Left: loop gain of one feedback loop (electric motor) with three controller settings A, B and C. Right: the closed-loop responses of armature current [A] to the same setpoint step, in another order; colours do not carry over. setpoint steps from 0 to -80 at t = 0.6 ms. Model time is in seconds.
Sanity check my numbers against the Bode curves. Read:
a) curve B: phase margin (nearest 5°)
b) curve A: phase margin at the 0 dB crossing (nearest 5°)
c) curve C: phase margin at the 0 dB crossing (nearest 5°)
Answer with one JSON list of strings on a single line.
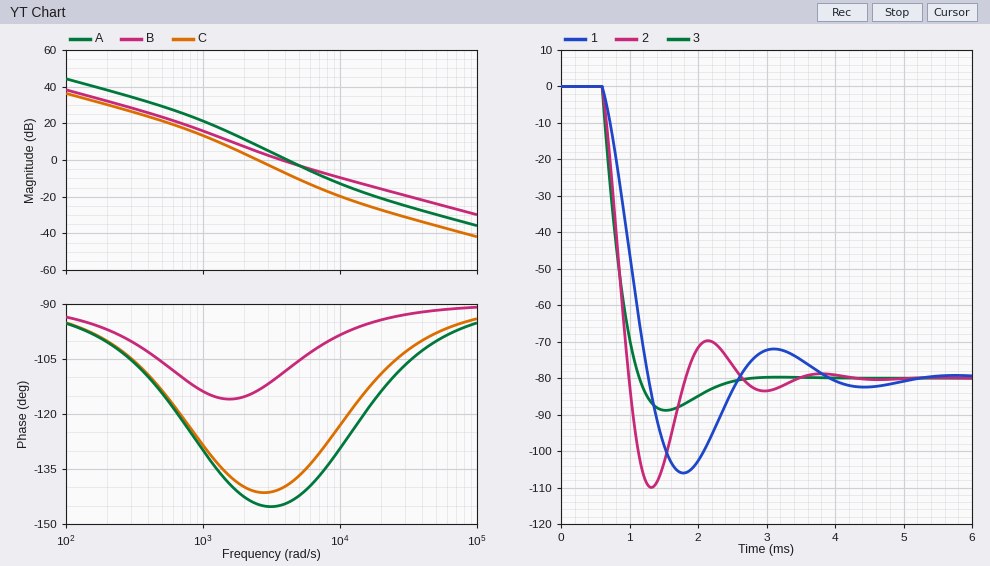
["70°", "35°", "40°"]
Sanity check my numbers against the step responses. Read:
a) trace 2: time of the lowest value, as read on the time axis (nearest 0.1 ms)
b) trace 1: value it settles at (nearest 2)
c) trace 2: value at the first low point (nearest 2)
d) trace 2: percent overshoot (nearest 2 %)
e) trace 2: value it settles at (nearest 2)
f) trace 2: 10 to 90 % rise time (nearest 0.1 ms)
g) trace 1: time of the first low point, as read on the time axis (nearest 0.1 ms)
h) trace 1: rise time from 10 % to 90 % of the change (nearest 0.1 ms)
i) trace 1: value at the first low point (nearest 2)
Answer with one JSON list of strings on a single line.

["1.3 ms", "-80", "-110", "38 %", "-80", "0.3 ms", "1.8 ms", "0.5 ms", "-106"]
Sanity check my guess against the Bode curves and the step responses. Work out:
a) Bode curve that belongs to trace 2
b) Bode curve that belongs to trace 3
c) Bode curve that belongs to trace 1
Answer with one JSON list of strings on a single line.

["A", "B", "C"]
